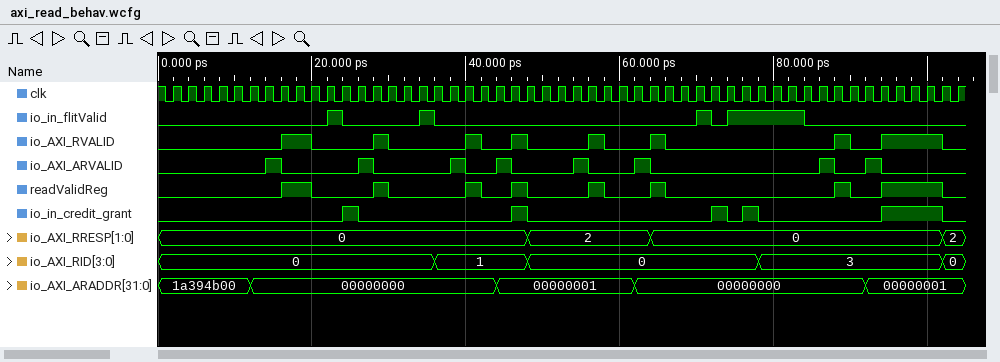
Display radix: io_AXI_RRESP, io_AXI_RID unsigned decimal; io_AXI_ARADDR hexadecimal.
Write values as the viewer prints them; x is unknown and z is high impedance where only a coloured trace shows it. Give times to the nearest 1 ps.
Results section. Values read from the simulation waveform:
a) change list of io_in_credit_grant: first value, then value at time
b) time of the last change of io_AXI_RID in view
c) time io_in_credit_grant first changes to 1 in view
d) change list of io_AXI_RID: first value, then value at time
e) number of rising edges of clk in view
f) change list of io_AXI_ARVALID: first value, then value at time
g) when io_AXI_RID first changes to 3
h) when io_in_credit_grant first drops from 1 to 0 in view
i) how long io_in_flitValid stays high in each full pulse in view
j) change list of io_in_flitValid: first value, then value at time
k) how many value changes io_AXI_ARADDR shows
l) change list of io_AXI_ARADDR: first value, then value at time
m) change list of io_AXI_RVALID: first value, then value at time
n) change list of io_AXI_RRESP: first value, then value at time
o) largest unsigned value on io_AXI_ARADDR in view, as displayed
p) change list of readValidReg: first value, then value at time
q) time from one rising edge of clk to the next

0, 1 at 24 ps, 0 at 26 ps, 1 at 46 ps, 0 at 48 ps, 1 at 72 ps, 0 at 74 ps, 1 at 76 ps, 0 at 78 ps, 1 at 94 ps, 0 at 102 ps
102 ps
24 ps
0, 1 at 36 ps, 0 at 48 ps, 3 at 78 ps, 0 at 102 ps
52
0, 1 at 14 ps, 0 at 16 ps, 1 at 26 ps, 0 at 28 ps, 1 at 38 ps, 0 at 40 ps, 1 at 44 ps, 0 at 46 ps, 1 at 54 ps, 0 at 56 ps, 1 at 62 ps, 0 at 64 ps, 1 at 86 ps, 0 at 88 ps, 1 at 92 ps, 0 at 94 ps
78 ps
26 ps
2 ps, 2 ps, 2 ps, 10 ps
0, 1 at 22 ps, 0 at 24 ps, 1 at 34 ps, 0 at 36 ps, 1 at 70 ps, 0 at 72 ps, 1 at 74 ps, 0 at 84 ps
4
1a394b00, 00000000 at 12 ps, 00000001 at 44 ps, 00000000 at 62 ps, 00000001 at 92 ps
0, 1 at 16 ps, 0 at 20 ps, 1 at 28 ps, 0 at 30 ps, 1 at 40 ps, 0 at 42 ps, 1 at 46 ps, 0 at 48 ps, 1 at 56 ps, 0 at 58 ps, 1 at 64 ps, 0 at 66 ps, 1 at 88 ps, 0 at 90 ps, 1 at 94 ps, 0 at 102 ps
0, 2 at 48 ps, 0 at 64 ps, 2 at 102 ps
1a394b00
0, 1 at 16 ps, 0 at 20 ps, 1 at 28 ps, 0 at 30 ps, 1 at 40 ps, 0 at 42 ps, 1 at 46 ps, 0 at 48 ps, 1 at 56 ps, 0 at 58 ps, 1 at 64 ps, 0 at 66 ps, 1 at 88 ps, 0 at 90 ps, 1 at 94 ps, 0 at 102 ps
2 ps
